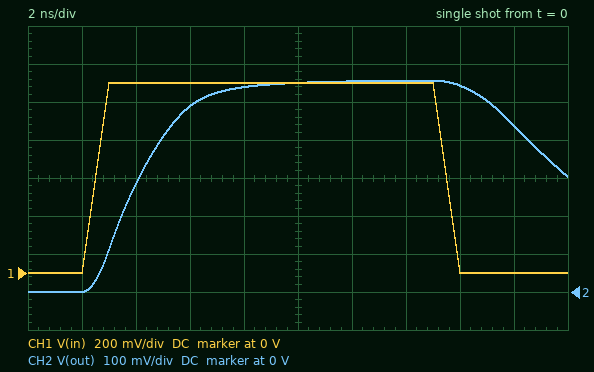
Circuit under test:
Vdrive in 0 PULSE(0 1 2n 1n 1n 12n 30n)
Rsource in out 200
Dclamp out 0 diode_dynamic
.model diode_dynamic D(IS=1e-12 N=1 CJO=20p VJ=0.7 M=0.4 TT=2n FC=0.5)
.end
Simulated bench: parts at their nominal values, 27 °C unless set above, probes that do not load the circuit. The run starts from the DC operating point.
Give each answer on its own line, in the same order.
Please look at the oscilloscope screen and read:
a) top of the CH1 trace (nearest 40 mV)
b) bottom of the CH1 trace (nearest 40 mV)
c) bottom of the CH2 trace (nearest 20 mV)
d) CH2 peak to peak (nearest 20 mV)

1.00 V
0 V
0 V
560 mV
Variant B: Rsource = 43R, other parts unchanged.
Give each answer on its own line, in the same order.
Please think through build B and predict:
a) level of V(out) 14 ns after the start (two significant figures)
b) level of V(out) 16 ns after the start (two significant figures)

590 mV
580 mV
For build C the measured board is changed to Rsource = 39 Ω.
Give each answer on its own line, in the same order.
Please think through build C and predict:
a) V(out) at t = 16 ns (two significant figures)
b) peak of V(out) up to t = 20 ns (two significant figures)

580 mV
600 mV
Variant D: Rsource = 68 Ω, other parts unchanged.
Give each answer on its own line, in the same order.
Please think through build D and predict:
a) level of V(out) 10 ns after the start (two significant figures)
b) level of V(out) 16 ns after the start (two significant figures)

580 mV
570 mV
